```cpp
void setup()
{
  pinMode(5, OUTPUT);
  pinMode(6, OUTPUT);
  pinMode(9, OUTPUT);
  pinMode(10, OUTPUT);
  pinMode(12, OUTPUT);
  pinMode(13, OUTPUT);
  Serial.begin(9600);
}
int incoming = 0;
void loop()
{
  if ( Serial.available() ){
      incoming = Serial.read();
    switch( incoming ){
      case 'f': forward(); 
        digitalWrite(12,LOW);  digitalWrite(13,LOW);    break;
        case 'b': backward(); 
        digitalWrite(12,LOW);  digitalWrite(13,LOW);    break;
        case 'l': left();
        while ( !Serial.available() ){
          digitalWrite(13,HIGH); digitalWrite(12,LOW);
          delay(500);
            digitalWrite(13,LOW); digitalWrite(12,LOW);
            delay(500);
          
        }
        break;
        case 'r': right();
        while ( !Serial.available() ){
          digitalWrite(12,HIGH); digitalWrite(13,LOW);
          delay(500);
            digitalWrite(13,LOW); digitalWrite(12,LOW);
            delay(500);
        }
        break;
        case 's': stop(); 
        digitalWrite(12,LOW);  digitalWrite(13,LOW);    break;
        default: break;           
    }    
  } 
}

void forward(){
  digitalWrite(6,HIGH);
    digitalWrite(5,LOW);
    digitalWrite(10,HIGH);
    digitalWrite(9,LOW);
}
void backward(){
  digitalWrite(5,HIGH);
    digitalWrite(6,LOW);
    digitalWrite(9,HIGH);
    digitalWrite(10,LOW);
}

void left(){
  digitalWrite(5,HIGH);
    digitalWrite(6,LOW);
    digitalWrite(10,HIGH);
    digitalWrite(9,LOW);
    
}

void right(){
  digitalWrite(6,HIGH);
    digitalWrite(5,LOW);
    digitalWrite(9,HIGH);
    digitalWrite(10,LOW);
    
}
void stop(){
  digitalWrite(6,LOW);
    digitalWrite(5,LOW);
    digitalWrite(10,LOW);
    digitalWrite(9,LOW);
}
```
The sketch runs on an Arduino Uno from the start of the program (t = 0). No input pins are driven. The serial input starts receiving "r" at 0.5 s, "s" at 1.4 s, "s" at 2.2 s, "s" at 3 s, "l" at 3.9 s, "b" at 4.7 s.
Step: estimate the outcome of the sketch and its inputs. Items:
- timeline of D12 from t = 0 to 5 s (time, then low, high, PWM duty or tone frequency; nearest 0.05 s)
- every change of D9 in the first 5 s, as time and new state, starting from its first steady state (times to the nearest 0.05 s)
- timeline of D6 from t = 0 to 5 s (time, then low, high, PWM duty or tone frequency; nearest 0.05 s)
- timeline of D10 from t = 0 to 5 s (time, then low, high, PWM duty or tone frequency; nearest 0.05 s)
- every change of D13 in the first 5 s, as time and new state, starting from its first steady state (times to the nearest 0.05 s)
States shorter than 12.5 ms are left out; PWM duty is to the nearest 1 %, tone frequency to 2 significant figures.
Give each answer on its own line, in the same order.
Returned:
0 s low; 0.5 s high; 1 s low
0 s low; 0.5 s high; 1.5 s low; 4.9 s high
0 s low; 0.5 s high; 1.5 s low
0 s low; 3.9 s high; 4.9 s low
0 s low; 3.9 s high; 4.4 s low
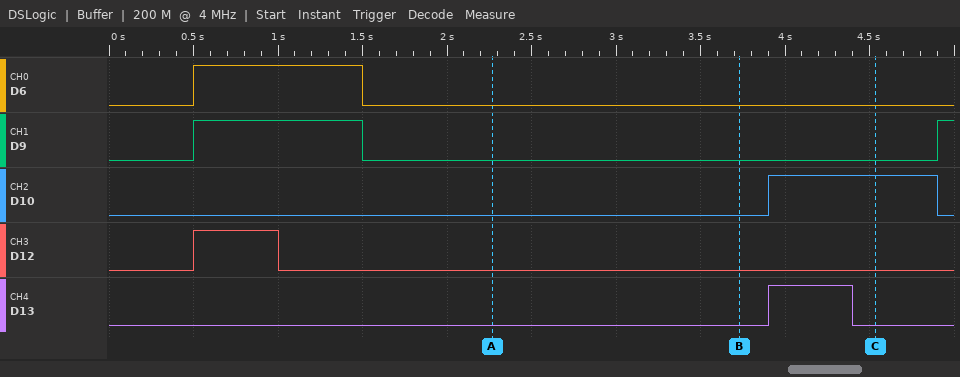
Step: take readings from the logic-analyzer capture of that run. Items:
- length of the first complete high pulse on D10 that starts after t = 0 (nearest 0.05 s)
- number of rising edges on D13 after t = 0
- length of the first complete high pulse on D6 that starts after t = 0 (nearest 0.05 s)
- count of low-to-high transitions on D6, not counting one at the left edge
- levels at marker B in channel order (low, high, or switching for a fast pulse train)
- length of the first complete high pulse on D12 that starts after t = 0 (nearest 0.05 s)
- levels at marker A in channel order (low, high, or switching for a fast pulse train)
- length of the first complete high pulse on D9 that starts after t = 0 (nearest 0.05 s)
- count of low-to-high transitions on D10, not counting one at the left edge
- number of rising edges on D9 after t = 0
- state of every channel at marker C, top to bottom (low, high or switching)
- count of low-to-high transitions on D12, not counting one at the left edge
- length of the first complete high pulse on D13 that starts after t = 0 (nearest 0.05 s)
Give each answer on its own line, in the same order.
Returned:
1.00 s
1
1.00 s
1
D6 low, D9 low, D10 low, D12 low, D13 low
0.50 s
D6 low, D9 low, D10 low, D12 low, D13 low
1.00 s
1
2
D6 low, D9 low, D10 high, D12 low, D13 low
1
0.50 s
